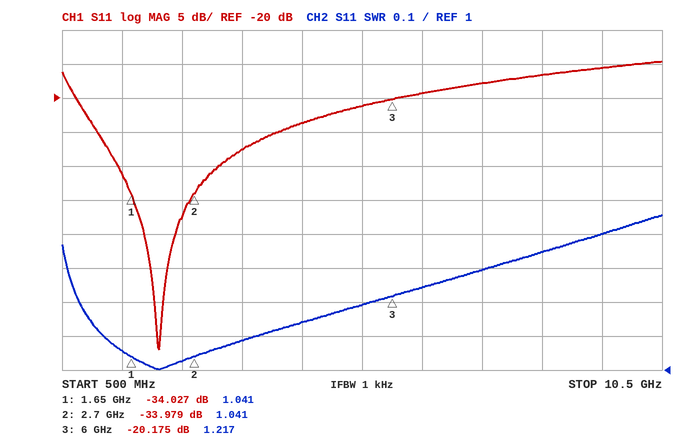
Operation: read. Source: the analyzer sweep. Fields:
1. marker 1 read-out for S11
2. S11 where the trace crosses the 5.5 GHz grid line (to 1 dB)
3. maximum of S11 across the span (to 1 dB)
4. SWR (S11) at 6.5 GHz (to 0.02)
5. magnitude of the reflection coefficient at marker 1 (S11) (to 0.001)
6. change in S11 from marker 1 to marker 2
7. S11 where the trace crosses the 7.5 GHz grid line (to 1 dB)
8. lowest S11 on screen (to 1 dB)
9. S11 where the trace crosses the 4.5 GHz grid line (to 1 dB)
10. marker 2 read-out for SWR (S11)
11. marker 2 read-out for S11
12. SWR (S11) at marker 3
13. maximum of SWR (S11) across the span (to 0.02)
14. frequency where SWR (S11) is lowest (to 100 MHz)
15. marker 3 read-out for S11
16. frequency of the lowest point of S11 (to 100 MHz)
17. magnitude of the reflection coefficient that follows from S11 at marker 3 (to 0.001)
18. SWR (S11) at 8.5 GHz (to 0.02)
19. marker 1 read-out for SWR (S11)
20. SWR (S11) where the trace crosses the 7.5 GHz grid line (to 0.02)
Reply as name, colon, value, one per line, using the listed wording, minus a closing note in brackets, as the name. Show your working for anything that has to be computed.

marker 1 read-out for S11: -34.027 dB
S11 where the trace crosses the 5.5 GHz grid line: -21 dB
maximum of S11 across the span: -15 dB
SWR (S11) at 6.5 GHz: 1.24
magnitude of the reflection coefficient at marker 1 (S11): 10^(-34.027/20) ≈ 0.020
change in S11 from marker 1 to marker 2: -33.979 − (-34.027) = 0.048 dB
S11 where the trace crosses the 7.5 GHz grid line: -18 dB
lowest S11 on screen: -57 dB
S11 where the trace crosses the 4.5 GHz grid line: -24 dB
marker 2 read-out for SWR: 1.041
marker 2 read-out for S11: -33.979 dB
SWR (S11) at marker 3: 1.217
maximum of SWR (S11) across the span: 1.46
frequency where SWR (S11) is lowest: 2.1 GHz
marker 3 read-out for S11: -20.175 dB
frequency of the lowest point of S11: 2.1 GHz
magnitude of the reflection coefficient that follows from S11 at marker 3: 10^(-20.175/20) ≈ 0.098
SWR (S11) at 8.5 GHz: 1.34
marker 1 read-out for SWR: 1.041
SWR (S11) where the trace crosses the 7.5 GHz grid line: 1.30
